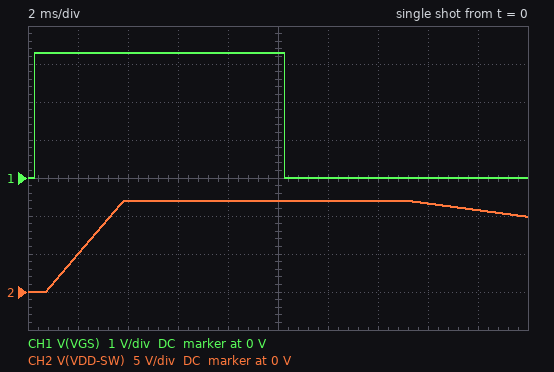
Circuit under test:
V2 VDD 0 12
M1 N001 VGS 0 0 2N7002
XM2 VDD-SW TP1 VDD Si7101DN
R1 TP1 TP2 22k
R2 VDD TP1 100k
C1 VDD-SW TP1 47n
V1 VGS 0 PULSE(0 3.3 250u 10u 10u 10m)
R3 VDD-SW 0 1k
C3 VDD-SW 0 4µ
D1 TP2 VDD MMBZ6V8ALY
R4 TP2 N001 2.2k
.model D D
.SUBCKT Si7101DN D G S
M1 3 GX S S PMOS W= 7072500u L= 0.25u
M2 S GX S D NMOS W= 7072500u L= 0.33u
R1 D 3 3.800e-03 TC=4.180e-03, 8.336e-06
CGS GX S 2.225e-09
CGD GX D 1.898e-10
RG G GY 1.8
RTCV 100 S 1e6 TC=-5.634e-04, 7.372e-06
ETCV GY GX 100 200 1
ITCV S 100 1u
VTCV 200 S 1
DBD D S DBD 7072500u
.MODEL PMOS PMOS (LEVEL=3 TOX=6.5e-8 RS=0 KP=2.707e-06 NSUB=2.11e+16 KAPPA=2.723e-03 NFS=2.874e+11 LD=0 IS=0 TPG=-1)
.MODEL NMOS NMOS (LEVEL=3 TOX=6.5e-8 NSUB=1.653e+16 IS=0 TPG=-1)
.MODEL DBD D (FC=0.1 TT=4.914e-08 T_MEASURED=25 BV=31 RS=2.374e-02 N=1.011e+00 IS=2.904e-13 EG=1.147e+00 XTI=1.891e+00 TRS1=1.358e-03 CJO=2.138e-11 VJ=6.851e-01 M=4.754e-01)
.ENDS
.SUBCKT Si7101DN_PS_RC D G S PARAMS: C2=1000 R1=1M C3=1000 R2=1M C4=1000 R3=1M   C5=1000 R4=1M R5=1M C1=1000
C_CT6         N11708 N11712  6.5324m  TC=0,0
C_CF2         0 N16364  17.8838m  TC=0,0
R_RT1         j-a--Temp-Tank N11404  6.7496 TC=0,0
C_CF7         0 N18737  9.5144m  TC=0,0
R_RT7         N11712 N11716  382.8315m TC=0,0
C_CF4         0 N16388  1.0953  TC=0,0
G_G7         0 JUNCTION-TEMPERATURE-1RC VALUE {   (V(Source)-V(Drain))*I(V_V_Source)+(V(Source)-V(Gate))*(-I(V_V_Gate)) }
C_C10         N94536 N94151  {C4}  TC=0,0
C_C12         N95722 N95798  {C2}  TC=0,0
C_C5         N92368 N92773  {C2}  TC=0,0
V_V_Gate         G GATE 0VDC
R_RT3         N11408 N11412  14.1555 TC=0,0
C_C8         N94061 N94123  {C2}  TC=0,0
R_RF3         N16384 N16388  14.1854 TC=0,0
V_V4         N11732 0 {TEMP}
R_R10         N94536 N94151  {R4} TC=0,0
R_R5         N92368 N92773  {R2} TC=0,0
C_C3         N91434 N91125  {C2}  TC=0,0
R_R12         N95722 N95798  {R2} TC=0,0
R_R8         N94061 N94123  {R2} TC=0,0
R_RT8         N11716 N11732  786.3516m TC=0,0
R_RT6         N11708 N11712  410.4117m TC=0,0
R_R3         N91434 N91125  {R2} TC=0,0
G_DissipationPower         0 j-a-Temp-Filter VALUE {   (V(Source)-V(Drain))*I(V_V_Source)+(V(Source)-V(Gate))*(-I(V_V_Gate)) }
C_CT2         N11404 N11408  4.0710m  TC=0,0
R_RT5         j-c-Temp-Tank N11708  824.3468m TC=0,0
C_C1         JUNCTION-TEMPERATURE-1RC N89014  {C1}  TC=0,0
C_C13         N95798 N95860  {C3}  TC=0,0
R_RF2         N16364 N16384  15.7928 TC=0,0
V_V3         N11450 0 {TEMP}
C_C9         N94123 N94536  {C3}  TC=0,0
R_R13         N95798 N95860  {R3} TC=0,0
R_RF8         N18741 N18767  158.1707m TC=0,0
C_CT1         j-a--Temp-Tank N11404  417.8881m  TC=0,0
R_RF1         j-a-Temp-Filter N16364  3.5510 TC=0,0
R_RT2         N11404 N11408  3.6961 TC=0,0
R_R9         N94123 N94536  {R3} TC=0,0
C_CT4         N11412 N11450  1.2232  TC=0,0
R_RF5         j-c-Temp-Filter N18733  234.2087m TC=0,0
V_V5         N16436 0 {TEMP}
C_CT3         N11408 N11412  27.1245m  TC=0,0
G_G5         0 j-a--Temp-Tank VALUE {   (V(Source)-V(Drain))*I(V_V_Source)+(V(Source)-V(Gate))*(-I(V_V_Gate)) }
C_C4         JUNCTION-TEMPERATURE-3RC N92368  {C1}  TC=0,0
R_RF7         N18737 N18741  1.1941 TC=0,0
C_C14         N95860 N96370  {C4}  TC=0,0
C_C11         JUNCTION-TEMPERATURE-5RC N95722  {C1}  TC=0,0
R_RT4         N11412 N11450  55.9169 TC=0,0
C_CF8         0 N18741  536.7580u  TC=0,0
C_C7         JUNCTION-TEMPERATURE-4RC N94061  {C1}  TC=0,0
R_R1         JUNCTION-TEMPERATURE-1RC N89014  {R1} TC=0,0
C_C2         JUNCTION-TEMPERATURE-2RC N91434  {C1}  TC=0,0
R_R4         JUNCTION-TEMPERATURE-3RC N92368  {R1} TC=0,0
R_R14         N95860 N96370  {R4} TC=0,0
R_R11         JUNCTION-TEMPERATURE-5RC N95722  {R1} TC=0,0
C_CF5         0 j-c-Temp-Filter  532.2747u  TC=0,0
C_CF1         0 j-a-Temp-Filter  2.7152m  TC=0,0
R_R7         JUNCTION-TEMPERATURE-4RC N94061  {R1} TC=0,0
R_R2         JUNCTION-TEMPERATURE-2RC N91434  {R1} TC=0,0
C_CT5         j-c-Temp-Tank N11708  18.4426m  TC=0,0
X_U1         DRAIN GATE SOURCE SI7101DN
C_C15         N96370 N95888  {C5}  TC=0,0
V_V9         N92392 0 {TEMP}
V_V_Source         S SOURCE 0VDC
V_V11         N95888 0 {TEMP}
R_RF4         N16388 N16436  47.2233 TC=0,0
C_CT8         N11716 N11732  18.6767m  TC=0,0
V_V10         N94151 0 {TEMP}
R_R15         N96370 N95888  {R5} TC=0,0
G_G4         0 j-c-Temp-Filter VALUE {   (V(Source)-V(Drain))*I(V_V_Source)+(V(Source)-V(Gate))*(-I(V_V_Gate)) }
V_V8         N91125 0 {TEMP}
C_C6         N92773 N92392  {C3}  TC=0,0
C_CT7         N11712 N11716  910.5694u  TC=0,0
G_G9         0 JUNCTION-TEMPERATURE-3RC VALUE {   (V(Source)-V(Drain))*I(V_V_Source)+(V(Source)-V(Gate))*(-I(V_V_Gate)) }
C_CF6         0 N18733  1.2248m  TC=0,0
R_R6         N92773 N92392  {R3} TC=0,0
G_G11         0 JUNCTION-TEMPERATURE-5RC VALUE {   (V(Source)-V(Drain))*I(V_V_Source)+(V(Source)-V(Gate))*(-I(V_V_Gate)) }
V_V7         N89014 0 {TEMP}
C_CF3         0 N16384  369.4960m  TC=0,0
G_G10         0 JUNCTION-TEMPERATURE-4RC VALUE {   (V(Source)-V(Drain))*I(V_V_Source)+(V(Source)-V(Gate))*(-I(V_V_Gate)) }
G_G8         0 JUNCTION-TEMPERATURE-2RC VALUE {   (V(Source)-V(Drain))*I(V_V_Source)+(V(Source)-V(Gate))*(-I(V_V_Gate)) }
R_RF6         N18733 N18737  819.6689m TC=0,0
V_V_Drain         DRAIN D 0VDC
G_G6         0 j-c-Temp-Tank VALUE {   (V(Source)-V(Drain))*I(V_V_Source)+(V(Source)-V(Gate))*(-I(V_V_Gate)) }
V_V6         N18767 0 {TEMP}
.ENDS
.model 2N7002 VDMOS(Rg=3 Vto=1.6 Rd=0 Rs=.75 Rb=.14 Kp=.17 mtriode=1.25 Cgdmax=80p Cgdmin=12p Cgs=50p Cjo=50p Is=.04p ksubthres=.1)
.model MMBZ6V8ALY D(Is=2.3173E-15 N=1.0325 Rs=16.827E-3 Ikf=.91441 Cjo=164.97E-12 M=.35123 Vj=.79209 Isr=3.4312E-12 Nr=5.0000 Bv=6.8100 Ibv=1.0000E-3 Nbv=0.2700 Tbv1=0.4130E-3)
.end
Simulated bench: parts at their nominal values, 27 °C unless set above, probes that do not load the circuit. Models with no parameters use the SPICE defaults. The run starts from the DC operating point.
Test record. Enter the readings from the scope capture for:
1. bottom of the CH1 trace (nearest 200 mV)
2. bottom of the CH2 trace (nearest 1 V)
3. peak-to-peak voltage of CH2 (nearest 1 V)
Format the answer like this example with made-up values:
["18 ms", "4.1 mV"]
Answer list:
["0 V", "0 V", "12 V"]
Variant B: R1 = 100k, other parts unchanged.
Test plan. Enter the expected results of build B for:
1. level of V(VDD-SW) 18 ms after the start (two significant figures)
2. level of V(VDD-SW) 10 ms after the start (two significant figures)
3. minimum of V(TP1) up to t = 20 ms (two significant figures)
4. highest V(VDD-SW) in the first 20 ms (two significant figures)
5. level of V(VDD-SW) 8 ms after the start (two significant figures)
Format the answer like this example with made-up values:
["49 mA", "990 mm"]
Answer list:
["1.3 V", "4.0 V", "9.9 V", "4.1 V", "2.9 V"]
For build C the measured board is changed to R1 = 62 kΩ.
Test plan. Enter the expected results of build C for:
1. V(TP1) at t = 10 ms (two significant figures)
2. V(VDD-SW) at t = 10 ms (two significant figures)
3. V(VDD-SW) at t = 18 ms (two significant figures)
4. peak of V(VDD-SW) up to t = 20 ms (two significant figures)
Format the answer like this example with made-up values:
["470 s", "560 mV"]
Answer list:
["9.8 V", "9.3 V", "6.3 V", "9.6 V"]
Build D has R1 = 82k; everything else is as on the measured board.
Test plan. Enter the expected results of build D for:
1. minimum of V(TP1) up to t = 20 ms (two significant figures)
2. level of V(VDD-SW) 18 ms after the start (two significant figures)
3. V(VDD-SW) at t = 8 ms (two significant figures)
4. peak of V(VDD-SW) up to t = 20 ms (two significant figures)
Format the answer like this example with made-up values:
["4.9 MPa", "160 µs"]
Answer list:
["9.9 V", "2.9 V", "4.4 V", "6.1 V"]
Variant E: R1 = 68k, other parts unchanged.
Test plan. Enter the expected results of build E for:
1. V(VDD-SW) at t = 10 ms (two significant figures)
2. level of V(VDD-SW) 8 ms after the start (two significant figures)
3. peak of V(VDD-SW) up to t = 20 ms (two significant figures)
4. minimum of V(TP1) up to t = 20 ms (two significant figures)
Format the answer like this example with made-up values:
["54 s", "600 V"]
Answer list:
["8.0 V", "6.1 V", "8.3 V", "9.8 V"]
